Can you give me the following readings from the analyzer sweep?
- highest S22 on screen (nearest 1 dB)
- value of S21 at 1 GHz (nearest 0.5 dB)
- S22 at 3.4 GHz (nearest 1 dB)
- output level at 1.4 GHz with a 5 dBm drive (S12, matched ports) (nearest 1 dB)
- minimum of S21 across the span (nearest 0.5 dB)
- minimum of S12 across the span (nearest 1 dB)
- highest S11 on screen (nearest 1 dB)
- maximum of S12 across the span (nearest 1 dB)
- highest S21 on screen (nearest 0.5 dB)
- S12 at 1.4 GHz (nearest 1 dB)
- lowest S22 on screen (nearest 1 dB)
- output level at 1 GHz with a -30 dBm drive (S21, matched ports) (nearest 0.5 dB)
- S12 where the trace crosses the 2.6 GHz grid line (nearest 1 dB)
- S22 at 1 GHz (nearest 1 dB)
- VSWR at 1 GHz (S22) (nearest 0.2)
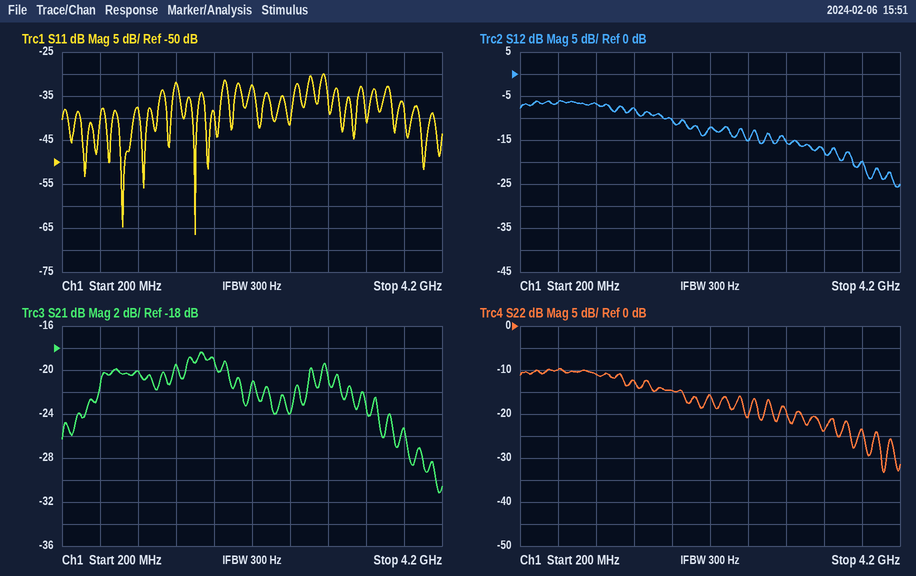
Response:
-10 dB
-20.0 dB
-24 dB
-3 dBm
-31.0 dB
-26 dB
-30 dB
-6 dB
-18.5 dB
-8 dB
-33 dB
-50.0 dBm
-15 dB
-11 dB
1.8
